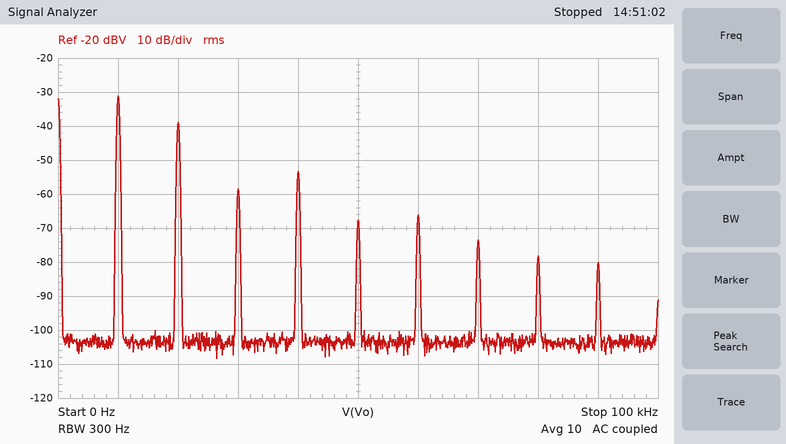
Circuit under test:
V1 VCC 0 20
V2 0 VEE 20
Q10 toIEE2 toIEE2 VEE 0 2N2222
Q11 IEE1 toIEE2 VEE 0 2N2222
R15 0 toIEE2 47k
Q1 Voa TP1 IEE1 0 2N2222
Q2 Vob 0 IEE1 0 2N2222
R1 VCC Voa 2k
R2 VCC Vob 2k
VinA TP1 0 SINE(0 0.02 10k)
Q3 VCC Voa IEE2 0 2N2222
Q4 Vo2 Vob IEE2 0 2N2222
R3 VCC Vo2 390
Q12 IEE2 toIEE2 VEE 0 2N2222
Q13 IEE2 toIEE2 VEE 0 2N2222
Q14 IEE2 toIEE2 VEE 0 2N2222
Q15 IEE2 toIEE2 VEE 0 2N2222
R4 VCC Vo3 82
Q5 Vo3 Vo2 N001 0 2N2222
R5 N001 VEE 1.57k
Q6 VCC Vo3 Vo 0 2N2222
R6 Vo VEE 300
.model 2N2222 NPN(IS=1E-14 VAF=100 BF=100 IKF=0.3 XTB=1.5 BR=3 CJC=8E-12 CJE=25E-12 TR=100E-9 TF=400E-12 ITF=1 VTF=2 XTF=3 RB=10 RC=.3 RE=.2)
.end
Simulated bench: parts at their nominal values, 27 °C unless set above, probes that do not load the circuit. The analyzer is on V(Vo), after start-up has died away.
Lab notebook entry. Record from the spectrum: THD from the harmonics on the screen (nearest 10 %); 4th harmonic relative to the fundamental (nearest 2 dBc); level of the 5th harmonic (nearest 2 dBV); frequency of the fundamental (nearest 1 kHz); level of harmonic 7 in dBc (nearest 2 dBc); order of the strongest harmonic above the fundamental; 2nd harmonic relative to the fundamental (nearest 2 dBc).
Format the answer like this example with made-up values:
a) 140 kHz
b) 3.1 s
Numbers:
a) 40 %
b) -22 dBc
c) -68 dBV
d) 10 kHz
e) -42 dBc
f) 2
g) -8 dBc
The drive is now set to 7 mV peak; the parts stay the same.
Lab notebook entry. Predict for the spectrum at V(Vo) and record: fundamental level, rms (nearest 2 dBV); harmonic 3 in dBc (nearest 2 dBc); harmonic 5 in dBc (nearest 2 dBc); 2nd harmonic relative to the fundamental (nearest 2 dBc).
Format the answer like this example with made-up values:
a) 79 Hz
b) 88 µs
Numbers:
a) -38 dBV
b) -30 dBc
c) -48 dBc
d) -12 dBc
